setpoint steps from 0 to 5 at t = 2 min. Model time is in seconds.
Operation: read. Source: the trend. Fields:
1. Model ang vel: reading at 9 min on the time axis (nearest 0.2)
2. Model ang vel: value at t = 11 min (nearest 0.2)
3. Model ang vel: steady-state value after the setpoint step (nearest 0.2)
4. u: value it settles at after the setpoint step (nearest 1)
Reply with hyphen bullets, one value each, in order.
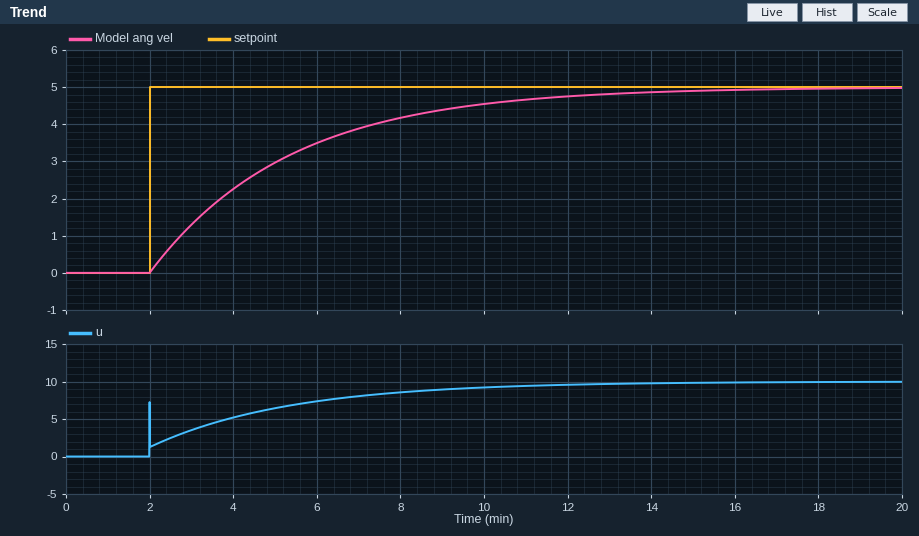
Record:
- 4.4
- 4.6
- 5.0
- 10
